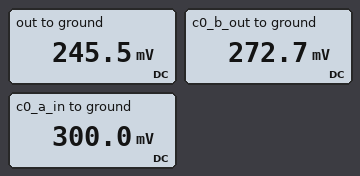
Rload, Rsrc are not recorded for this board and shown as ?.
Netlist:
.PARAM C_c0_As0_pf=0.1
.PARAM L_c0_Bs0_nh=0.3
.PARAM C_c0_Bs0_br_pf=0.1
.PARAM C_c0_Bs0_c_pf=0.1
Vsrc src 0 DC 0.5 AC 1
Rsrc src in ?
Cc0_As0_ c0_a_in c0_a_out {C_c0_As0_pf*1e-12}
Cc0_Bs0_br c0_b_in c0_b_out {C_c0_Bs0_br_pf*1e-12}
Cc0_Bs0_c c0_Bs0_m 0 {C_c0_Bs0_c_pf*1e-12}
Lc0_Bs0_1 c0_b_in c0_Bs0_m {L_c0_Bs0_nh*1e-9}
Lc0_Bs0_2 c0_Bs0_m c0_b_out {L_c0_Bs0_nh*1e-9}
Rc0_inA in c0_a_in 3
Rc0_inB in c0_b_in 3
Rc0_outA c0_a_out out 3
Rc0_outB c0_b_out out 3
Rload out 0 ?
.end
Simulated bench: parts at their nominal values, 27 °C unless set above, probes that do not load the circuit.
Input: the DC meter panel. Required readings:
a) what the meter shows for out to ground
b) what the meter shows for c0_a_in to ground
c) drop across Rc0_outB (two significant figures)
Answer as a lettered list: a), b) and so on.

a) 245.5 mV
b) 300.0 mV
c) 27 mV
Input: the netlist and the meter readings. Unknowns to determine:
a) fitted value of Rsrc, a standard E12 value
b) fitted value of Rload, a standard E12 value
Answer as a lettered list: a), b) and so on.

a) 22 Ω
b) 27 Ω
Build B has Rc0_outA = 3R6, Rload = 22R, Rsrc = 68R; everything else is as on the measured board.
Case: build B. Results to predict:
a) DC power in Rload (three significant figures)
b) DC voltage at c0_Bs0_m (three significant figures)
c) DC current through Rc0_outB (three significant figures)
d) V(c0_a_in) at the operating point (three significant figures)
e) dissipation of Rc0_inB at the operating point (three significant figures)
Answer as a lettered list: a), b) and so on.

a) 597 µW
b) 130 mV
c) 5.21 mA
d) 146 mV
e) 81.4 µW
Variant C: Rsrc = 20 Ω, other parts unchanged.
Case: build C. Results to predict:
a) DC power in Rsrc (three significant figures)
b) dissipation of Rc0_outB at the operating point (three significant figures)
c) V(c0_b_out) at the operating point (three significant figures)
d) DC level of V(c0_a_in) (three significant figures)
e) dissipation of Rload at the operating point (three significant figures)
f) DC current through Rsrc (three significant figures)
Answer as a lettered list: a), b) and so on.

a) 1.78 mW
b) 267 µW
c) 283 mV
d) 311 mV
e) 2.40 mW
f) 9.43 mA
